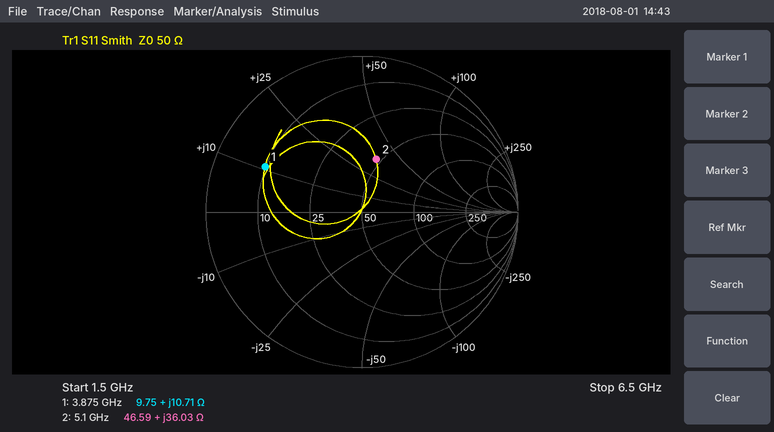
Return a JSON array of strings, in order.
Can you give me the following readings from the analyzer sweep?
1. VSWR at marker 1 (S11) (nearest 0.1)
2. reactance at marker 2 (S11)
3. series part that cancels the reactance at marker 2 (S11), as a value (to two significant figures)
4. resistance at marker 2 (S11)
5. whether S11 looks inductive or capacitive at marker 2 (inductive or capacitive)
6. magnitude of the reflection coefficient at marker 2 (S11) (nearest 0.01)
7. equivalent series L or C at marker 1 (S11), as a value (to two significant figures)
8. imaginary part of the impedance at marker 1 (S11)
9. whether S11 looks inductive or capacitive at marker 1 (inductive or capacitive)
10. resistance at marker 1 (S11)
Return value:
["5.4", "+36.03 Ω", "870 fF", "46.59 Ω", "inductive", "0.35", "440 pH", "+10.71 Ω", "inductive", "9.75 Ω"]
